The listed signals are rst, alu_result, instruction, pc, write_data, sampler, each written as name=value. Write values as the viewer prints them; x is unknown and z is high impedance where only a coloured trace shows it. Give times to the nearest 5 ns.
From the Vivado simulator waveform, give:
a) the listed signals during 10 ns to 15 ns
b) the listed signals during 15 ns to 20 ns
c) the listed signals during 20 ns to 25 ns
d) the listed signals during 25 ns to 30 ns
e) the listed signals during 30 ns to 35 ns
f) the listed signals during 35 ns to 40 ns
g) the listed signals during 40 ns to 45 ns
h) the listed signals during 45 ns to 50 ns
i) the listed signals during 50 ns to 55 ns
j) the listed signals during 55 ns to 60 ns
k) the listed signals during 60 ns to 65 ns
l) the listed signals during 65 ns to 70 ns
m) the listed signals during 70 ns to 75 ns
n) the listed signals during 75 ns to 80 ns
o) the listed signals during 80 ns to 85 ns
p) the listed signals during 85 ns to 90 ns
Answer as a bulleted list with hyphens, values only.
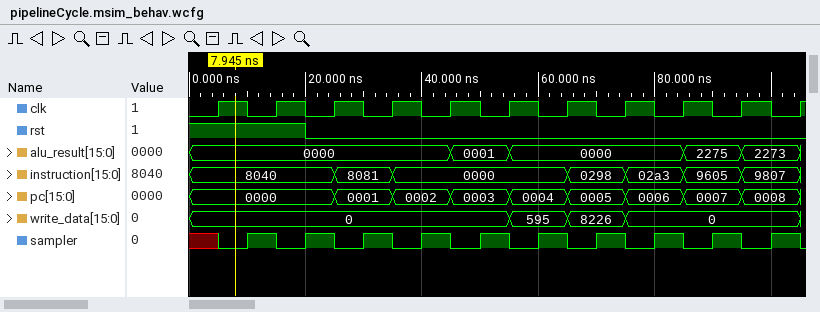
- rst=1, alu_result=0000, instruction=8040, pc=0000, write_data=0, sampler=1
- rst=1, alu_result=0000, instruction=8040, pc=0000, write_data=0, sampler=0
- rst=0, alu_result=0000, instruction=8040, pc=0000, write_data=0, sampler=1
- rst=0, alu_result=0000, instruction=8081, pc=0001, write_data=0, sampler=0
- rst=0, alu_result=0000, instruction=8081, pc=0001, write_data=0, sampler=1
- rst=0, alu_result=0000, instruction=0000, pc=0002, write_data=0, sampler=0
- rst=0, alu_result=0000, instruction=0000, pc=0002, write_data=0, sampler=1
- rst=0, alu_result=0001, instruction=0000, pc=0003, write_data=0, sampler=0
- rst=0, alu_result=0001, instruction=0000, pc=0003, write_data=0, sampler=1
- rst=0, alu_result=0000, instruction=0000, pc=0004, write_data=595, sampler=0
- rst=0, alu_result=0000, instruction=0000, pc=0004, write_data=595, sampler=1
- rst=0, alu_result=0000, instruction=0298, pc=0005, write_data=8226, sampler=0
- rst=0, alu_result=0000, instruction=0298, pc=0005, write_data=8226, sampler=1
- rst=0, alu_result=0000, instruction=02a3, pc=0006, write_data=0, sampler=0
- rst=0, alu_result=0000, instruction=02a3, pc=0006, write_data=0, sampler=1
- rst=0, alu_result=2275, instruction=9605, pc=0007, write_data=0, sampler=0
